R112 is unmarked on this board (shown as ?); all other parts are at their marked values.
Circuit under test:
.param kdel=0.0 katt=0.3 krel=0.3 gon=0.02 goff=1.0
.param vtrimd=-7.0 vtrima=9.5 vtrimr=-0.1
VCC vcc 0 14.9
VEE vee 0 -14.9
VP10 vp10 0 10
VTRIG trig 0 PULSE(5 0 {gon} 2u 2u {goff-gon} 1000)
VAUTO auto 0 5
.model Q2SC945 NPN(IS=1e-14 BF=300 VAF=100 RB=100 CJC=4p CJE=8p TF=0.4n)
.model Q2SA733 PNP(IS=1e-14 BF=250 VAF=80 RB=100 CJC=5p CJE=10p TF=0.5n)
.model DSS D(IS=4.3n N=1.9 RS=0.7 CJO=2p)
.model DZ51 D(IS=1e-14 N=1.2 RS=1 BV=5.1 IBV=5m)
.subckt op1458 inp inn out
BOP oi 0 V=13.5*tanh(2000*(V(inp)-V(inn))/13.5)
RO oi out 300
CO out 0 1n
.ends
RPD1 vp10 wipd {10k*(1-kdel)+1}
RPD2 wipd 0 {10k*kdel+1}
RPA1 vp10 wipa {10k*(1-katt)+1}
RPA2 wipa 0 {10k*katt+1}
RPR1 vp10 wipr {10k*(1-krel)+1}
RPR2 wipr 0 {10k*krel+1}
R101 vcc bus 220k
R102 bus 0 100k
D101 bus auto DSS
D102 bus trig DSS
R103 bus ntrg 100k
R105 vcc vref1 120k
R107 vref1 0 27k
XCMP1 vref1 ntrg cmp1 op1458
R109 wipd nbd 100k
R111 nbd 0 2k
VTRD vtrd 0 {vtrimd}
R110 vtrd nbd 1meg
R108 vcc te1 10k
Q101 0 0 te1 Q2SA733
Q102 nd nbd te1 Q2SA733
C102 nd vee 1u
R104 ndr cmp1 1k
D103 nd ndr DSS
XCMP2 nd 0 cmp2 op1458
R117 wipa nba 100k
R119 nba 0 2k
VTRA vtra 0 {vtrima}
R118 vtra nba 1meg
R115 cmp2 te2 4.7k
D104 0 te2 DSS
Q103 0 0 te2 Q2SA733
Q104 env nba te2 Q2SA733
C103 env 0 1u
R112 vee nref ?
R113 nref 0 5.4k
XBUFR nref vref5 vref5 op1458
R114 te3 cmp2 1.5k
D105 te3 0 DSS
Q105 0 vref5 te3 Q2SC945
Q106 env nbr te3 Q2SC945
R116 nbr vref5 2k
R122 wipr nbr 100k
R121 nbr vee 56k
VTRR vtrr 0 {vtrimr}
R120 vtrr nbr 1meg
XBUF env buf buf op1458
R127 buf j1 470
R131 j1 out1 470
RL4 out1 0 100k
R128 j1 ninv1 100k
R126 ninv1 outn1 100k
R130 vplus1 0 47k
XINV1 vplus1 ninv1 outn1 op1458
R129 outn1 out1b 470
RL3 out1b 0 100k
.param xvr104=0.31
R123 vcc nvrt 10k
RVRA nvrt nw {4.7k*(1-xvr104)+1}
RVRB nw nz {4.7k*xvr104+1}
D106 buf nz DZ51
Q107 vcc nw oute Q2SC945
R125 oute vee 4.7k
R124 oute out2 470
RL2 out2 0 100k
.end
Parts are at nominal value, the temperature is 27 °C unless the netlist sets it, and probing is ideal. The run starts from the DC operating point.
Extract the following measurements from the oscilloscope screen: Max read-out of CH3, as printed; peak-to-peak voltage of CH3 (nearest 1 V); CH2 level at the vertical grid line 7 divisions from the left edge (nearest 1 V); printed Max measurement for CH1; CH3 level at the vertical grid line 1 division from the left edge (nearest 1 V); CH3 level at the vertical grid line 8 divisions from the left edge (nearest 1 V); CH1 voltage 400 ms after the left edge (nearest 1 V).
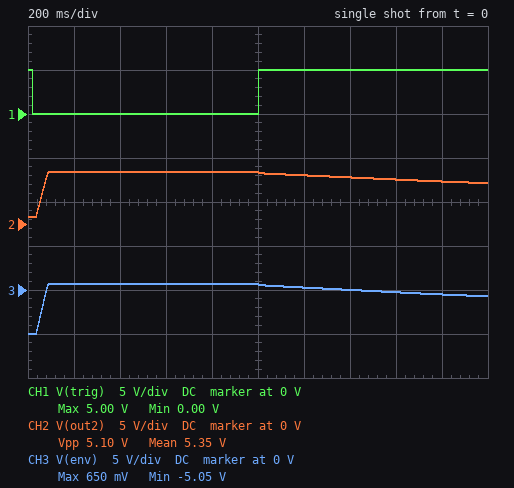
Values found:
650 mV
6 V
5 V
5.00 V
1 V
0 V
0 V
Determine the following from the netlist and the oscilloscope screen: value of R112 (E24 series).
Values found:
13 kΩ
